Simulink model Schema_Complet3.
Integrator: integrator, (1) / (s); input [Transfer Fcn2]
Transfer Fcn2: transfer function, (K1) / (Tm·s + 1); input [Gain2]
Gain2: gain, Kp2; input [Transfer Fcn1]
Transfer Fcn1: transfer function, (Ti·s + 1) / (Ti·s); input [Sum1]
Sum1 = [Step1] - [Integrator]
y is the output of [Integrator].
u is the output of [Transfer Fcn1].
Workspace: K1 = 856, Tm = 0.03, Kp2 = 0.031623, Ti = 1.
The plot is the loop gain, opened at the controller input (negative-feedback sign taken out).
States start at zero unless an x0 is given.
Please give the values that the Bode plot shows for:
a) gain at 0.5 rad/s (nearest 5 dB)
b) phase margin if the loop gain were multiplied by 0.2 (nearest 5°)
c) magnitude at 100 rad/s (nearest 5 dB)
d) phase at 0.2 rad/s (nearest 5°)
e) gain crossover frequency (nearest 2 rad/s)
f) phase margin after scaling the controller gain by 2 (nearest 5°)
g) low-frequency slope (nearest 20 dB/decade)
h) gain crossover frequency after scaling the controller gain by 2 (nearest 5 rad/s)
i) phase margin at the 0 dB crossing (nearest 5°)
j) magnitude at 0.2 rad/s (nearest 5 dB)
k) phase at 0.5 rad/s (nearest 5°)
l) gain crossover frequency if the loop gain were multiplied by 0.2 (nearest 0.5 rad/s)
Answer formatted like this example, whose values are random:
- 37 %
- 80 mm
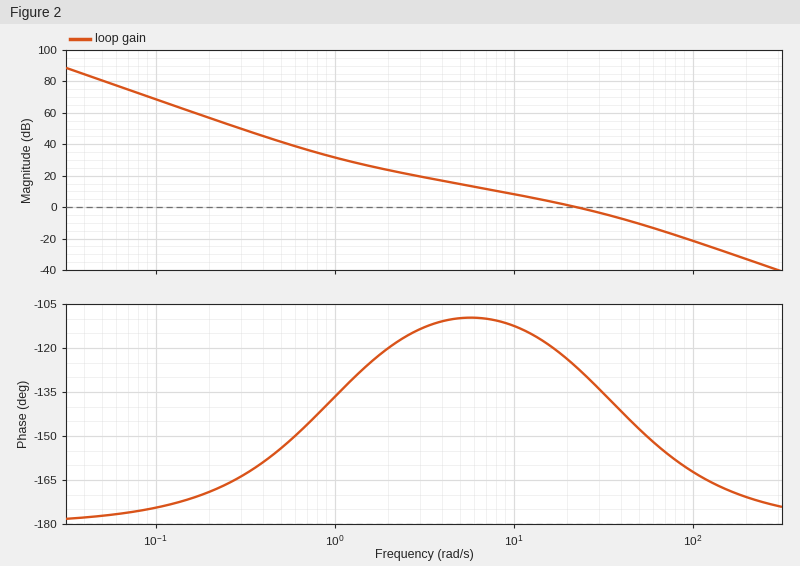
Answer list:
- 40 dB
- 70°
- -20 dB
- -170°
- 22 rad/s
- 40°
- -40 dB/decade
- 35 rad/s
- 55°
- 55 dB
- -155°
- 5.5 rad/s
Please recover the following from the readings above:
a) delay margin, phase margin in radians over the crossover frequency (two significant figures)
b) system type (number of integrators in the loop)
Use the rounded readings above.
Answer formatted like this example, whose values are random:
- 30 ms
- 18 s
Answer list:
- 0.044 s
- 2
